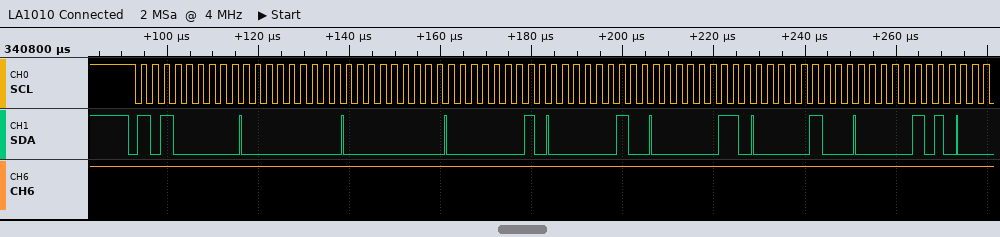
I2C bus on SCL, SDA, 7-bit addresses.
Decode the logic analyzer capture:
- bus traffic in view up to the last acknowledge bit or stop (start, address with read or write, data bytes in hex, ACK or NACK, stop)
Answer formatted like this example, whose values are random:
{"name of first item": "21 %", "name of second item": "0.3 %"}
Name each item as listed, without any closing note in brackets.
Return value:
{"bus traffic in view up to the last acknowledge bit or stop": "start, address 50 write ACK, 00 ACK, 00 ACK, 01 ACK, 02 ACK, 03 ACK, 04 ACK, 05 ACK"}
